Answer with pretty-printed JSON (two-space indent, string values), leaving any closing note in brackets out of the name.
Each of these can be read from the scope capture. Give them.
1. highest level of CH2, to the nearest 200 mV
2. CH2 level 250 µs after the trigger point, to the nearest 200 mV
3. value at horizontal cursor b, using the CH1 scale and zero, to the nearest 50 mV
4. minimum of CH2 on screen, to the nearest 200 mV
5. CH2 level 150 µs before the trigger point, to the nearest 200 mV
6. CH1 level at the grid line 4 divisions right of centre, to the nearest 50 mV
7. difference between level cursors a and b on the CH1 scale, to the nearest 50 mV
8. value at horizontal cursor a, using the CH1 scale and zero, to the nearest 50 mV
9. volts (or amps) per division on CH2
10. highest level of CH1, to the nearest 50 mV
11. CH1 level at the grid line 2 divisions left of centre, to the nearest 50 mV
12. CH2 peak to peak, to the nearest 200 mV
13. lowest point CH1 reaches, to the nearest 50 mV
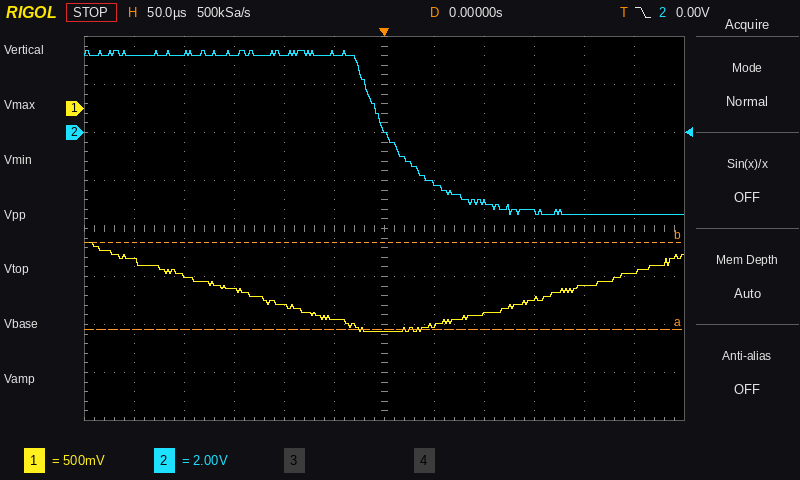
{
  "highest level of CH2, to the nearest 200 mV": "3.4 V",
  "CH2 level 250 µs after the trigger point, to the nearest 200 mV": "-3.4 V",
  "value at horizontal cursor b, using the CH1 scale and zero, to the nearest 50 mV": "-1.40 V",
  "minimum of CH2 on screen, to the nearest 200 mV": "-3.4 V",
  "CH2 level 150 µs before the trigger point, to the nearest 200 mV": "3.2 V",
  "CH1 level at the grid line 4 divisions right of centre, to the nearest 50 mV": "-1.85 V",
  "difference between level cursors a and b on the CH1 scale, to the nearest 50 mV": "900 mV",
  "value at horizontal cursor a, using the CH1 scale and zero, to the nearest 50 mV": "-2.30 V",
  "volts (or amps) per division on CH2": "2 V",
  "highest level of CH1, to the nearest 50 mV": "-1.40 V",
  "CH1 level at the grid line 2 divisions left of centre, to the nearest 50 mV": "-2.05 V",
  "CH2 peak to peak, to the nearest 200 mV": "6.8 V",
  "lowest point CH1 reaches, to the nearest 50 mV": "-2.30 V"
}
